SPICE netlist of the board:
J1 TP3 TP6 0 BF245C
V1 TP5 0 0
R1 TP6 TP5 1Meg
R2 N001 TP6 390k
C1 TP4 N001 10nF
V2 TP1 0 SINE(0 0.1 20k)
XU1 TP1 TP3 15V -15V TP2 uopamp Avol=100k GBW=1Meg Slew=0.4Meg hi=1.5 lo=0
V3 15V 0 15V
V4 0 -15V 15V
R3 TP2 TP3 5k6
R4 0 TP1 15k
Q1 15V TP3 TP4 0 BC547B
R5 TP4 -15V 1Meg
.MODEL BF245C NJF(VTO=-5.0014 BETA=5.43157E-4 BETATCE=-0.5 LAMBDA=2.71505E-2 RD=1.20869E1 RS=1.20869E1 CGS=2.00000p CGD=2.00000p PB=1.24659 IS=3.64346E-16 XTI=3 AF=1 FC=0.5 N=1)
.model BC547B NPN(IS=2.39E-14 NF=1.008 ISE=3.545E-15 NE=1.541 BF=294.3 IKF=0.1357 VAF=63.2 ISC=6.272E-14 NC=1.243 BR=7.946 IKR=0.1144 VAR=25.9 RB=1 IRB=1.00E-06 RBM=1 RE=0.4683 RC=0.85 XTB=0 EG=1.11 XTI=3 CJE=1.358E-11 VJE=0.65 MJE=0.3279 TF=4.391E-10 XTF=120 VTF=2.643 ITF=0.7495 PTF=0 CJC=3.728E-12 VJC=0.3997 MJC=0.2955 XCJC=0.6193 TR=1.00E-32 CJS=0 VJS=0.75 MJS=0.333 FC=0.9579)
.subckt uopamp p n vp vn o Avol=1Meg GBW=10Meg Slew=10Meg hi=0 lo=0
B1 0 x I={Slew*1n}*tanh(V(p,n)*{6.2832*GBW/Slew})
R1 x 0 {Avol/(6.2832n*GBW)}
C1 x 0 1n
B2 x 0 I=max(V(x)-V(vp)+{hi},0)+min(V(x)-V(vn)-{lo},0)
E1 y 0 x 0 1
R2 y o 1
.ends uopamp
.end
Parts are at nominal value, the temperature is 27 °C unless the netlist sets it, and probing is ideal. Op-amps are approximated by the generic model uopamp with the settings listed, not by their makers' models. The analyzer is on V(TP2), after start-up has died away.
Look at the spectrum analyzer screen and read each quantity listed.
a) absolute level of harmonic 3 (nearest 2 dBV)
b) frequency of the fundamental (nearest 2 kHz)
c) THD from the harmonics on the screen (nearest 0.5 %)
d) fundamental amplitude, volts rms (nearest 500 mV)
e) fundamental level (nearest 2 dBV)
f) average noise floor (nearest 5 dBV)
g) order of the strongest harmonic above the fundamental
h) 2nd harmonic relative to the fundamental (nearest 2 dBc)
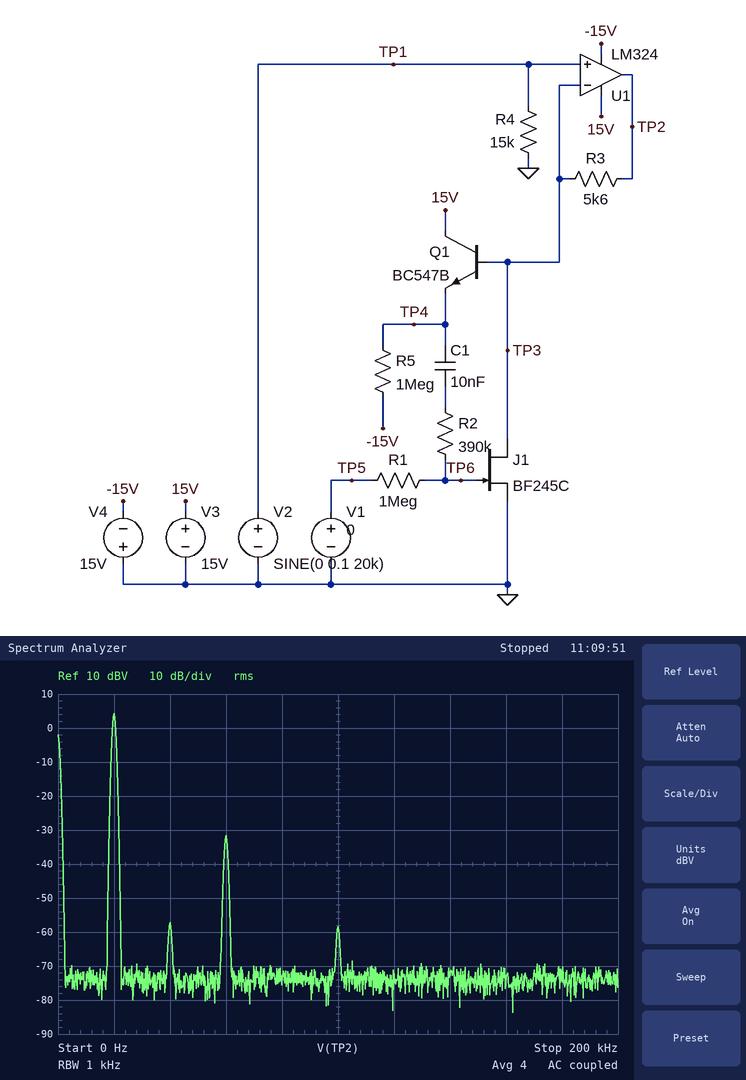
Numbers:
-32 dBV
20 kHz
1.5 %
1.5 V
4 dBV
-75 dBV
3
-62 dBc
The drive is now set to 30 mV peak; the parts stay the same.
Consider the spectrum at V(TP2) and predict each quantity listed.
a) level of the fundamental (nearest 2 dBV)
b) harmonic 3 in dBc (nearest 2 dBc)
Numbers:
-6 dBV
-58 dBc
